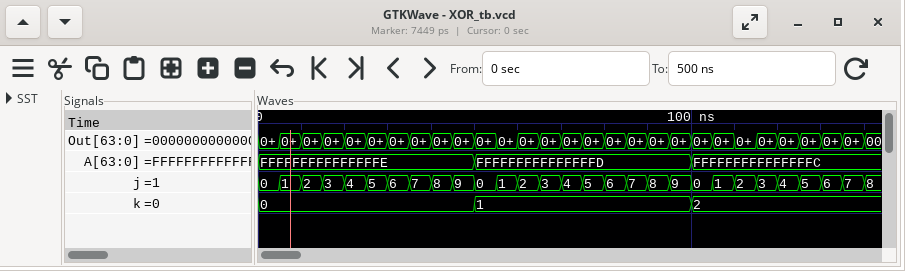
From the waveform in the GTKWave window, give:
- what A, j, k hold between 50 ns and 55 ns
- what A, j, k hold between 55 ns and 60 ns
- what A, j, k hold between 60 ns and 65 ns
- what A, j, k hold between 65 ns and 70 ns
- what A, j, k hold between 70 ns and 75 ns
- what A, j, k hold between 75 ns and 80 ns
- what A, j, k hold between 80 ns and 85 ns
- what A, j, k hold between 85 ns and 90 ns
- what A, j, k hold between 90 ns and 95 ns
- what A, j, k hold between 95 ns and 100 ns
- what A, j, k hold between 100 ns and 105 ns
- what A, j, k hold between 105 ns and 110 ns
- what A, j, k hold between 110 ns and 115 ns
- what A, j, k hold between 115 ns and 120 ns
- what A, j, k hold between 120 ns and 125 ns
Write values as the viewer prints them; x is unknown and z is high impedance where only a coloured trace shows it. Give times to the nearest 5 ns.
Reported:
A=FFFFFFFFFFFFFFFD, j=0, k=1
A=FFFFFFFFFFFFFFFD, j=1, k=1
A=FFFFFFFFFFFFFFFD, j=2, k=1
A=FFFFFFFFFFFFFFFD, j=3, k=1
A=FFFFFFFFFFFFFFFD, j=4, k=1
A=FFFFFFFFFFFFFFFD, j=5, k=1
A=FFFFFFFFFFFFFFFD, j=6, k=1
A=FFFFFFFFFFFFFFFD, j=7, k=1
A=FFFFFFFFFFFFFFFD, j=8, k=1
A=FFFFFFFFFFFFFFFD, j=9, k=1
A=FFFFFFFFFFFFFFFC, j=0, k=2
A=FFFFFFFFFFFFFFFC, j=1, k=2
A=FFFFFFFFFFFFFFFC, j=2, k=2
A=FFFFFFFFFFFFFFFC, j=3, k=2
A=FFFFFFFFFFFFFFFC, j=4, k=2
